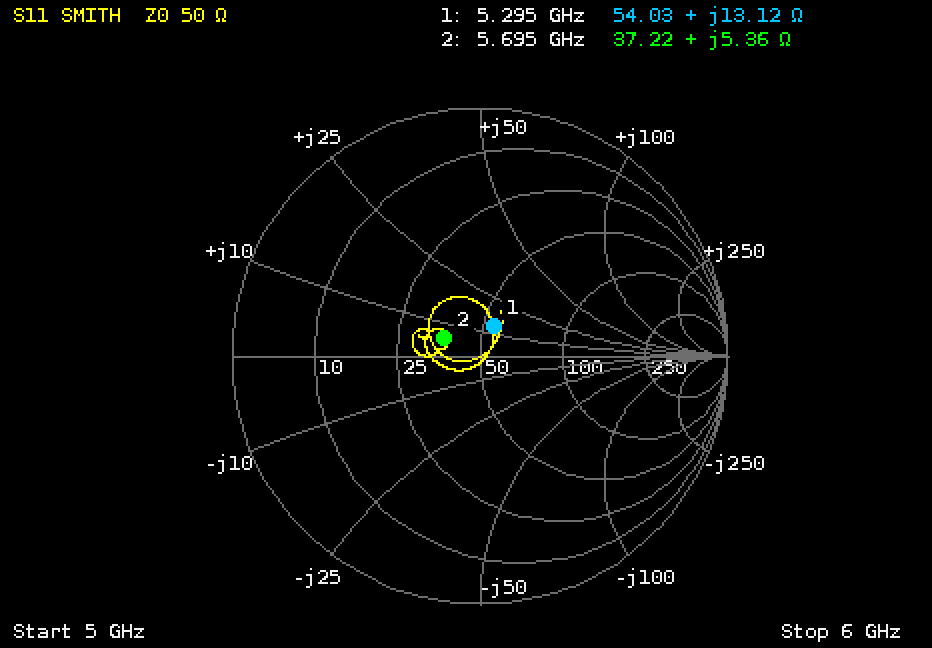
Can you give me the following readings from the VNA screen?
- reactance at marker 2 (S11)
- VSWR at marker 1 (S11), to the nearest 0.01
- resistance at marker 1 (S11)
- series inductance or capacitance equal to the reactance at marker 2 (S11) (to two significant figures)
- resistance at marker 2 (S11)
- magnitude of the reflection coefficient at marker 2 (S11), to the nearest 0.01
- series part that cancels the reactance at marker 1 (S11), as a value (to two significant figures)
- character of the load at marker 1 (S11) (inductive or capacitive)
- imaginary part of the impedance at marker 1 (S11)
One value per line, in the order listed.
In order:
+5.36 Ω
1.30
54.03 Ω
150 pH
37.22 Ω
0.16
2.3 pF
inductive
+13.12 Ω
